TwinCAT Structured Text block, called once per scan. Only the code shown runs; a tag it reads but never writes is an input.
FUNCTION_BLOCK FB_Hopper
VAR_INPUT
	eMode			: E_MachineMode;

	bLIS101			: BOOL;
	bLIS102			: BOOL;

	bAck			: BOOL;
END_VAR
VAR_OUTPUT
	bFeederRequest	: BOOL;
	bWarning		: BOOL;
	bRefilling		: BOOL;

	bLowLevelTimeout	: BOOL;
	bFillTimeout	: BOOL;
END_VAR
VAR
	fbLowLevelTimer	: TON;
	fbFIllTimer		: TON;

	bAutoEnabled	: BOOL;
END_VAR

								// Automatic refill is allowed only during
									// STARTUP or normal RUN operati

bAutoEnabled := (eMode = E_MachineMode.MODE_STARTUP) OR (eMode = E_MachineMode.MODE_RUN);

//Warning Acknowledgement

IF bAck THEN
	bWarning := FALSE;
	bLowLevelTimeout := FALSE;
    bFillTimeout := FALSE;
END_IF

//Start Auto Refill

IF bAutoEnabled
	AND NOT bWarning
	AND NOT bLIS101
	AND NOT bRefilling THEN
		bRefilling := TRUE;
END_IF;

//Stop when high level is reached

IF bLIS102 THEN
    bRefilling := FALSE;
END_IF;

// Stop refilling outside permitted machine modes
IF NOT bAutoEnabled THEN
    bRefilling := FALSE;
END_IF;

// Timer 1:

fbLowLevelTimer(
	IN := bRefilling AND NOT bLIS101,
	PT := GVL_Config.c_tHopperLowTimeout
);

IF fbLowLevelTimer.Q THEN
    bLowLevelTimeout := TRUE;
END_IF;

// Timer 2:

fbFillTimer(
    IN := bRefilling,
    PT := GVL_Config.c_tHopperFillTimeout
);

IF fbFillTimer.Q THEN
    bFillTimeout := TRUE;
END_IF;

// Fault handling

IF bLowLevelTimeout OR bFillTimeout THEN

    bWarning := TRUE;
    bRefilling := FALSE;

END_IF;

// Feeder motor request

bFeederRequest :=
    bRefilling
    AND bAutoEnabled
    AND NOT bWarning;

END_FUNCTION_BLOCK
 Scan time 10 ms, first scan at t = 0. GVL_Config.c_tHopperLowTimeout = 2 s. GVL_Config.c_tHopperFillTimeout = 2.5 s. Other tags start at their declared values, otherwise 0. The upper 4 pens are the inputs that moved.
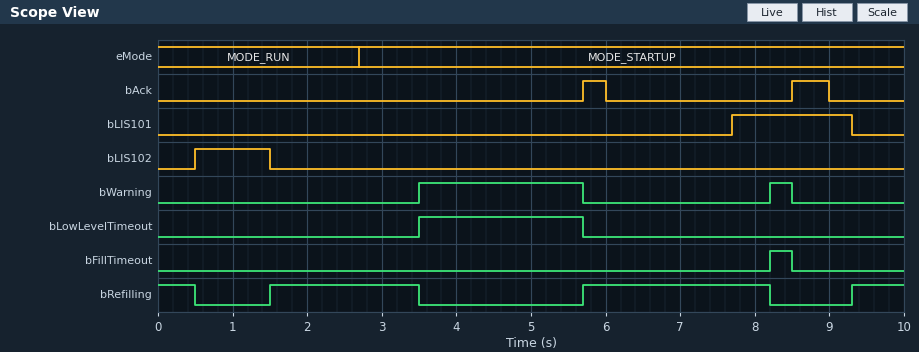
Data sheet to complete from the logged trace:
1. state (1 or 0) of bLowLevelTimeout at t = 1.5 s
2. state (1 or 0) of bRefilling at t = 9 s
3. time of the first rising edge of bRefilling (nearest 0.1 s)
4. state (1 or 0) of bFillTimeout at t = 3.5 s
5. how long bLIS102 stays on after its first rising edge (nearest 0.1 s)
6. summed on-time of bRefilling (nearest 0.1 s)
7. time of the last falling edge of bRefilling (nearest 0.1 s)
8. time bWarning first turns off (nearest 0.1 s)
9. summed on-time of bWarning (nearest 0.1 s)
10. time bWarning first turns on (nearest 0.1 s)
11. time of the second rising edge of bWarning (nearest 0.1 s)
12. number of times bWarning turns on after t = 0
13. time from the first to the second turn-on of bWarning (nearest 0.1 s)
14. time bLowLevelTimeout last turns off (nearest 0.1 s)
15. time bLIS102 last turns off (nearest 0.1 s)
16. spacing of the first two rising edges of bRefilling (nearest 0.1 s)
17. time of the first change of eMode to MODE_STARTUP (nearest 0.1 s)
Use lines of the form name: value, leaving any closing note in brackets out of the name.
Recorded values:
state (1 or 0) of bLowLevelTimeout at t = 1.5 s: 0
state (1 or 0) of bRefilling at t = 9 s: 0
time of the first rising edge of bRefilling: 1.5 s
state (1 or 0) of bFillTimeout at t = 3.5 s: 0
how long bLIS102 stays on after its first rising edge: 1.0 s
summed on-time of bRefilling: 5.7 s
time of the last falling edge of bRefilling: 8.2 s
time bWarning first turns off: 5.7 s
summed on-time of bWarning: 2.5 s
time bWarning first turns on: 3.5 s
time of the second rising edge of bWarning: 8.2 s
number of times bWarning turns on after t = 0: 2
time from the first to the second turn-on of bWarning: 4.7 s
time bLowLevelTimeout last turns off: 5.7 s
time bLIS102 last turns off: 1.5 s
spacing of the first two rising edges of bRefilling: 4.2 s
time of the first change of eMode to MODE_STARTUP: 2.7 s
